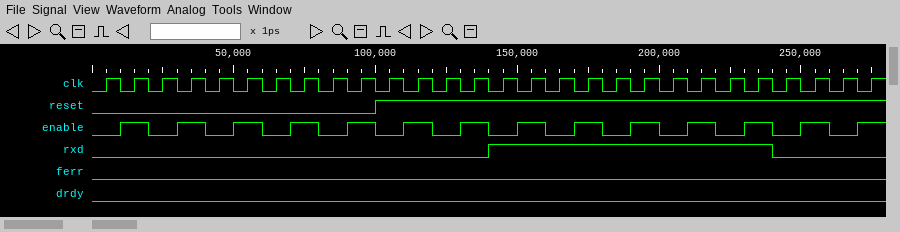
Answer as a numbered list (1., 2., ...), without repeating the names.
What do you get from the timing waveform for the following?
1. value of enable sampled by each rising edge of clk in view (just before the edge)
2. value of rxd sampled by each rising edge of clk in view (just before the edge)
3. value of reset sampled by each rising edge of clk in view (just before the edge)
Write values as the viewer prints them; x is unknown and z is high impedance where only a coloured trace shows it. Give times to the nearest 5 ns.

1. 0 1 0 1 0 1 0 1 0 1 0 1 0 1 0 1 0 1 0 1 0 1 0 1 0 1 0 1
2. 0 0 0 0 0 0 0 0 0 0 0 0 0 0 1 1 1 1 1 1 1 1 1 1 0 0 0 0
3. 0 0 0 0 0 0 0 0 0 0 1 1 1 1 1 1 1 1 1 1 1 1 1 1 1 1 1 1
